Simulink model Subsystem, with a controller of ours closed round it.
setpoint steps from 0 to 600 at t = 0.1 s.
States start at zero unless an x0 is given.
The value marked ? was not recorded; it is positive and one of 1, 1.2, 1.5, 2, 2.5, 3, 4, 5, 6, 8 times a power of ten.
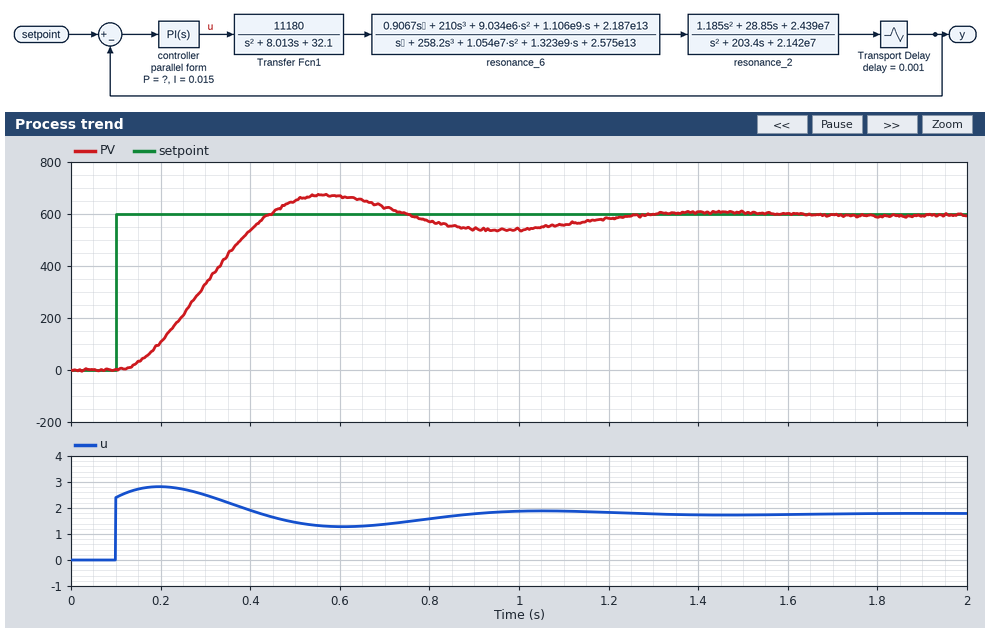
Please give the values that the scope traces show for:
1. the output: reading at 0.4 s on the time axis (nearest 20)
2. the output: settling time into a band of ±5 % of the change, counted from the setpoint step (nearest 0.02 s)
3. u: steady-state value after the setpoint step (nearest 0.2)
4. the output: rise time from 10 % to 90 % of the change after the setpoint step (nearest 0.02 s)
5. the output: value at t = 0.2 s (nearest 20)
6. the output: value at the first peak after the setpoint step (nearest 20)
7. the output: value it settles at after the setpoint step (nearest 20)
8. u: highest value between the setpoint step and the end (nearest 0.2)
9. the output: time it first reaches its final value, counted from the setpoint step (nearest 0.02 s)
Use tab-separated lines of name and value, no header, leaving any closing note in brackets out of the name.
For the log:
the output: reading at 0.4 s on the time axis	540
the output: settling time into a band of ±5 % of the change, counted from the setpoint step	1.04 s
u: steady-state value after the setpoint step	1.8
the output: rise time from 10 % to 90 % of the change after the setpoint step	0.22 s
the output: value at t = 0.2 s	100
the output: value at the first peak after the setpoint step	680
the output: value it settles at after the setpoint step	600
u: highest value between the setpoint step and the end	2.8
the output: time it first reaches its final value, counted from the setpoint step	0.34 s
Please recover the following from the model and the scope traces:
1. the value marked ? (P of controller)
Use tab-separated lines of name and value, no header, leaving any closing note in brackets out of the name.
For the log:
the value marked ?	0.004
